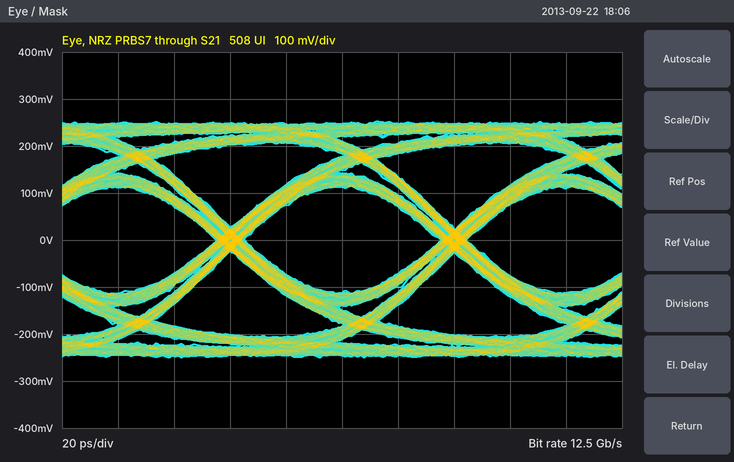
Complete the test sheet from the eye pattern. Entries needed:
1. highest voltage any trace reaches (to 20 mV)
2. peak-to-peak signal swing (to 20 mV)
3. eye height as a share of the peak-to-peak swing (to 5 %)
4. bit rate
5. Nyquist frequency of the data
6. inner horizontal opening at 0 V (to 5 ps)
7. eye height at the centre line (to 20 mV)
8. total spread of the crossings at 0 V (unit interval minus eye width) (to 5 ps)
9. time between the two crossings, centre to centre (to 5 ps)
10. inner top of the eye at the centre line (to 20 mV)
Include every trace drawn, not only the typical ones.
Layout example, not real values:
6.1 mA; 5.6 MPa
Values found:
260 mV; 500 mV; 45 %; 12.5 Gb/s; 6.25 GHz; 70 ps; 220 mV; 10 ps; 80 ps; 120 mV
